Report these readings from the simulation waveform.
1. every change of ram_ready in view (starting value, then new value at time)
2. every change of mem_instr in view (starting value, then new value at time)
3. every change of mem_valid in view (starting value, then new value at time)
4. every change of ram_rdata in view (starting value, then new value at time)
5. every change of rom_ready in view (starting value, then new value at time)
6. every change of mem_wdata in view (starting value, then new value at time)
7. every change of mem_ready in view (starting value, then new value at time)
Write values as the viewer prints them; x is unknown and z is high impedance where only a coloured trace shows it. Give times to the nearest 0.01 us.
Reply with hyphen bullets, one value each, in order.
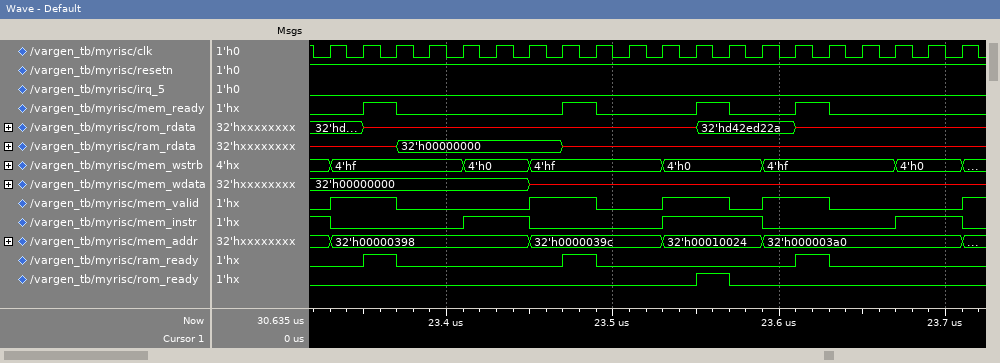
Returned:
- 0, 1 at 23.35 us, 0 at 23.37 us, 1 at 23.47 us, 0 at 23.49 us, 1 at 23.61 us, 0 at 23.63 us
- 1, 0 at 23.33 us, 1 at 23.41 us, 0 at 23.45 us, 1 at 23.53 us, 0 at 23.59 us, 1 at 23.67 us, 0 at 23.71 us
- 0, 1 at 23.33 us, 0 at 23.37 us, 1 at 23.45 us, 0 at 23.49 us, 1 at 23.53 us, 0 at 23.57 us, 1 at 23.59 us, 0 at 23.63 us, 1 at 23.71 us
- x, 32'h00000000 at 23.37 us, x at 23.47 us
- 0, 1 at 23.55 us, 0 at 23.57 us
- 32'h00000000, x at 23.45 us
- 0, 1 at 23.35 us, 0 at 23.37 us, 1 at 23.47 us, 0 at 23.49 us, 1 at 23.55 us, 0 at 23.57 us, 1 at 23.61 us, 0 at 23.63 us
